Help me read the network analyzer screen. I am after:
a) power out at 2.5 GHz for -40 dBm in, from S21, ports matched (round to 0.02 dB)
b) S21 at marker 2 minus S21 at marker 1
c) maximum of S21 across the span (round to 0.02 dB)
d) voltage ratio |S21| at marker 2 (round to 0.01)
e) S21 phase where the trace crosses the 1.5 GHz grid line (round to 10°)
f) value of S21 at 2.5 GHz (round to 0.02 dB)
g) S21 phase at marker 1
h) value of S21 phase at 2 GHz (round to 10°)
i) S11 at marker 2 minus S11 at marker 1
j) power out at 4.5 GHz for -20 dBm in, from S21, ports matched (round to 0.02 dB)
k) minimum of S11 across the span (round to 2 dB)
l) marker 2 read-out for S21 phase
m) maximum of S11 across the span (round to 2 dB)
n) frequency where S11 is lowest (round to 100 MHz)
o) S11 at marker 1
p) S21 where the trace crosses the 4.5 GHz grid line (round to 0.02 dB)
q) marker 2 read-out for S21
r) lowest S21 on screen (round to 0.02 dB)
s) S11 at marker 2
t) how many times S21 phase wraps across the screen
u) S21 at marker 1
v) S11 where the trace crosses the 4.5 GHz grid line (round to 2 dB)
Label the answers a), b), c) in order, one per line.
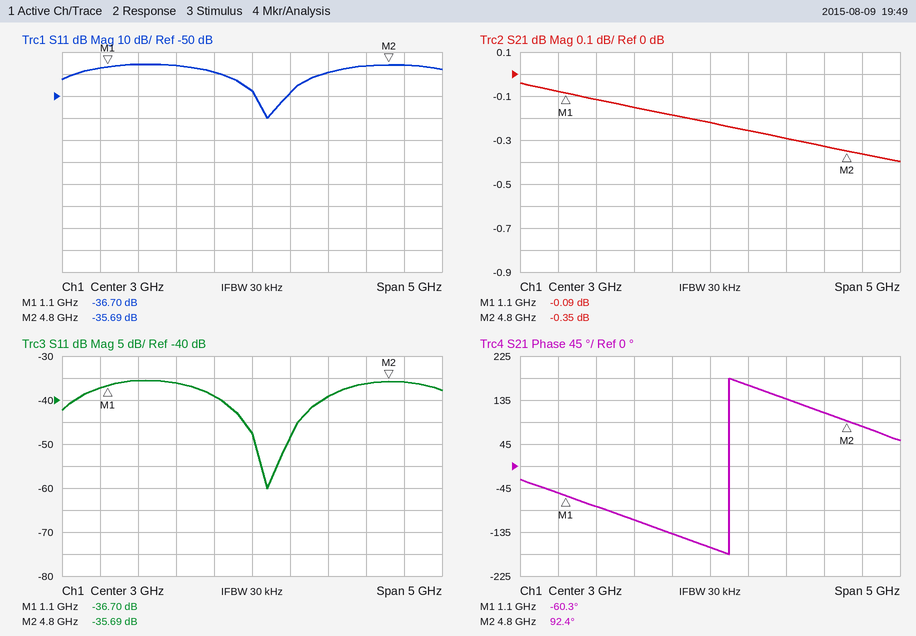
a) -40.18 dBm
b) -0.26 dB
c) -0.04 dB
d) 0.96
e) -80°
f) -0.18 dB
g) -60.3°
h) -110°
i) 1.01 dB
j) -20.32 dBm
k) -60 dB
l) 92.4°
m) -36 dB
n) 3.2 GHz
o) -36.70 dB
p) -0.32 dB
q) -0.35 dB
r) -0.40 dB
s) -35.69 dB
t) 1
u) -0.09 dB
v) -36 dB
